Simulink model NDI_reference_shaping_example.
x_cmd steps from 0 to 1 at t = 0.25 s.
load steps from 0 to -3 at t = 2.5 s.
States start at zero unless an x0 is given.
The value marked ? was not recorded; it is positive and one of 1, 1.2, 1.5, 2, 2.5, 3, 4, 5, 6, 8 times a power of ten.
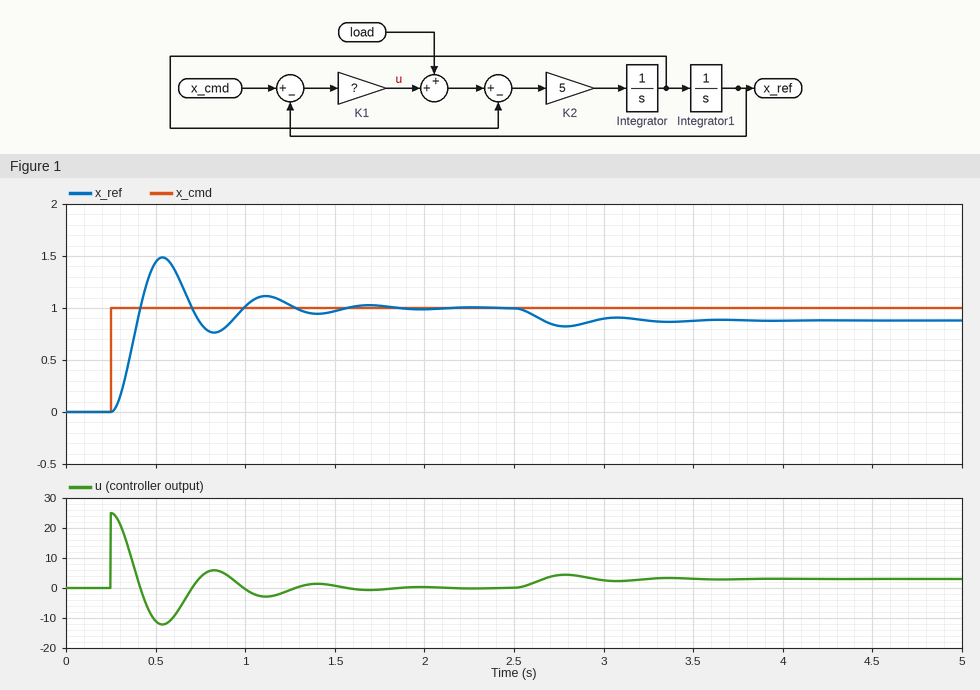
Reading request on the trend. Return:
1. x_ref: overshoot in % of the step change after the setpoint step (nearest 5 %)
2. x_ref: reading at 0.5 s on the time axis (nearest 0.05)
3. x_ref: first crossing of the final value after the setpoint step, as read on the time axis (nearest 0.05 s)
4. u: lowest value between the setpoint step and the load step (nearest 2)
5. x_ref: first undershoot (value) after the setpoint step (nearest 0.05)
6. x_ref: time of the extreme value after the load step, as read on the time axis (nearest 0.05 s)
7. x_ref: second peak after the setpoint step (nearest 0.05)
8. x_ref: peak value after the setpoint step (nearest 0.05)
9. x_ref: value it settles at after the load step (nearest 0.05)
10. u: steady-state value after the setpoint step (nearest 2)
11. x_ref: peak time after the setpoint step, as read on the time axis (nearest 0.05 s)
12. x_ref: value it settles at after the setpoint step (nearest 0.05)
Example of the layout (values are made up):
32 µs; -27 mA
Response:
50 %; 1.45; 0.40 s; -12; 0.75; 2.80 s; 1.10; 1.50; 0.90; 0; 0.55 s; 1.00
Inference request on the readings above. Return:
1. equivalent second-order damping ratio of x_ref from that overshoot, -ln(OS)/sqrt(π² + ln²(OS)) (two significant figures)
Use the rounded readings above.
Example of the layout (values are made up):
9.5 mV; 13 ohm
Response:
0.22
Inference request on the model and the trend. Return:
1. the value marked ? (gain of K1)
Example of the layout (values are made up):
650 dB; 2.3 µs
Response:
25
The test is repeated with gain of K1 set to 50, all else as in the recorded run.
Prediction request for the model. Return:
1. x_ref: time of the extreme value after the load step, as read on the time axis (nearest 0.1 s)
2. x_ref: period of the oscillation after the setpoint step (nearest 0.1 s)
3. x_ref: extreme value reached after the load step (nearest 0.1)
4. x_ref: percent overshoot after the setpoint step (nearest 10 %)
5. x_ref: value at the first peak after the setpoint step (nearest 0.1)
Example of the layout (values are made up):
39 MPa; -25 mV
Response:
2.7 s; 0.4 s; 0.9; 60 %; 1.6
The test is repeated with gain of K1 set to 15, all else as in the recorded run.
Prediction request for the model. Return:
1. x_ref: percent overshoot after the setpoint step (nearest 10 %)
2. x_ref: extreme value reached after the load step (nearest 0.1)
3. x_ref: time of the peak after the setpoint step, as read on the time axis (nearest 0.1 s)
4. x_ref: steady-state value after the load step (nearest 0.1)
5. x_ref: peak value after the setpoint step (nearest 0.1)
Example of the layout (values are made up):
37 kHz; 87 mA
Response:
40 %; 0.7; 0.6 s; 0.8; 1.4
